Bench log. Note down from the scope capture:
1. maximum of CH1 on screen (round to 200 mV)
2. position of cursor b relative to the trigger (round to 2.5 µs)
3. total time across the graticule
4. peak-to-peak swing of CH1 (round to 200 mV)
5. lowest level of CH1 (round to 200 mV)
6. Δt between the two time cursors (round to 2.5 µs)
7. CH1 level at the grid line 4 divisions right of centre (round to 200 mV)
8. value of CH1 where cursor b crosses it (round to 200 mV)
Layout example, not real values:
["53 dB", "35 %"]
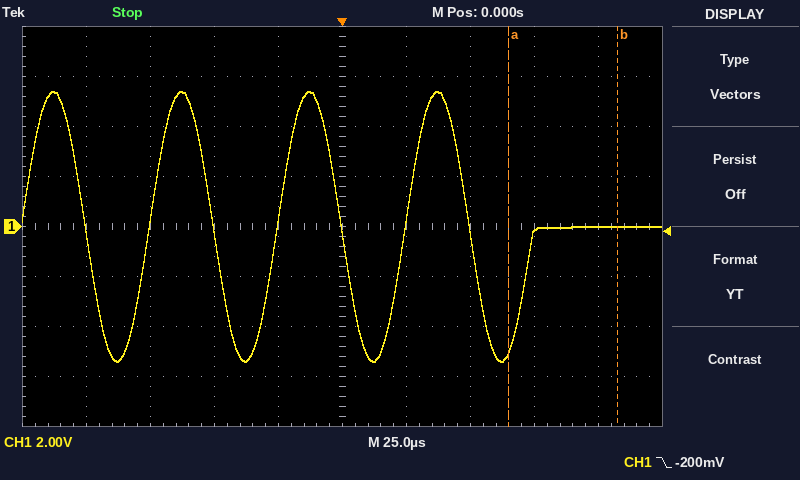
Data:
["5.4 V", "+107.5 µs", "250 µs", "10.8 V", "-5.4 V", "42.5 µs", "0.0 V", "0.0 V"]
